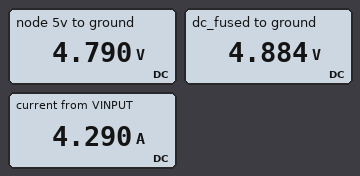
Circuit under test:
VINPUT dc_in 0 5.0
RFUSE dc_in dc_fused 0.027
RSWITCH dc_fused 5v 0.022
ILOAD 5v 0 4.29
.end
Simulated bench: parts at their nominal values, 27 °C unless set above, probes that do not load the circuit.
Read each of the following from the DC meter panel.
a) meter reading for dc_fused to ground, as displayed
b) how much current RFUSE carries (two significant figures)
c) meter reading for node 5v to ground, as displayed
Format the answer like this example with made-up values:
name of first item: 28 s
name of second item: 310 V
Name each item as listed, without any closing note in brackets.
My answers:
meter reading for dc_fused to ground, as displayed: 4.884 V
how much current RFUSE carries: 4.3 A
meter reading for node 5v to ground, as displayed: 4.790 V
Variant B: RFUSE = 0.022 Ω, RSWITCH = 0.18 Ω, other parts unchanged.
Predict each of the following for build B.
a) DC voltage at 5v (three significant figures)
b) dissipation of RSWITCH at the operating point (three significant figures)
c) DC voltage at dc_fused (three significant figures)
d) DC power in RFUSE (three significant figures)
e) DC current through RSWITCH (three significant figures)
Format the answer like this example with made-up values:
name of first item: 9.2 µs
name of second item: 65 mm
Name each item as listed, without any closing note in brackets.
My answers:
DC voltage at 5v: 4.13 V
dissipation of RSWITCH at the operating point: 3.31 W
DC voltage at dc_fused: 4.91 V
DC power in RFUSE: 405 mW
DC current through RSWITCH: 4.29 A
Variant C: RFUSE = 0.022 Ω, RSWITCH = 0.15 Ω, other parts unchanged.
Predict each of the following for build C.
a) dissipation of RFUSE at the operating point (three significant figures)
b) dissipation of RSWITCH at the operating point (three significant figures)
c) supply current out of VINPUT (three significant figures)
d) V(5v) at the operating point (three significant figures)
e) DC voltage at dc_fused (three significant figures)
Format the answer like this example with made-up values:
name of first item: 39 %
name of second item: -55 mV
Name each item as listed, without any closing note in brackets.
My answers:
dissipation of RFUSE at the operating point: 405 mW
dissipation of RSWITCH at the operating point: 2.76 W
supply current out of VINPUT: 4.29 A
V(5v) at the operating point: 4.26 V
DC voltage at dc_fused: 4.91 V
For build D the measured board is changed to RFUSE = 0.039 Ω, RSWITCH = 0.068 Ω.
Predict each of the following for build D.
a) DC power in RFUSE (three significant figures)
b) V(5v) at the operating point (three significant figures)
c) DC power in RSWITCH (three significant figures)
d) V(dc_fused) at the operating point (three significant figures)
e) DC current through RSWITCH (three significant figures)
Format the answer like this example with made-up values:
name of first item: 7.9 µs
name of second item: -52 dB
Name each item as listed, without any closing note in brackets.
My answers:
DC power in RFUSE: 718 mW
V(5v) at the operating point: 4.54 V
DC power in RSWITCH: 1.25 W
V(dc_fused) at the operating point: 4.83 V
DC current through RSWITCH: 4.29 A
